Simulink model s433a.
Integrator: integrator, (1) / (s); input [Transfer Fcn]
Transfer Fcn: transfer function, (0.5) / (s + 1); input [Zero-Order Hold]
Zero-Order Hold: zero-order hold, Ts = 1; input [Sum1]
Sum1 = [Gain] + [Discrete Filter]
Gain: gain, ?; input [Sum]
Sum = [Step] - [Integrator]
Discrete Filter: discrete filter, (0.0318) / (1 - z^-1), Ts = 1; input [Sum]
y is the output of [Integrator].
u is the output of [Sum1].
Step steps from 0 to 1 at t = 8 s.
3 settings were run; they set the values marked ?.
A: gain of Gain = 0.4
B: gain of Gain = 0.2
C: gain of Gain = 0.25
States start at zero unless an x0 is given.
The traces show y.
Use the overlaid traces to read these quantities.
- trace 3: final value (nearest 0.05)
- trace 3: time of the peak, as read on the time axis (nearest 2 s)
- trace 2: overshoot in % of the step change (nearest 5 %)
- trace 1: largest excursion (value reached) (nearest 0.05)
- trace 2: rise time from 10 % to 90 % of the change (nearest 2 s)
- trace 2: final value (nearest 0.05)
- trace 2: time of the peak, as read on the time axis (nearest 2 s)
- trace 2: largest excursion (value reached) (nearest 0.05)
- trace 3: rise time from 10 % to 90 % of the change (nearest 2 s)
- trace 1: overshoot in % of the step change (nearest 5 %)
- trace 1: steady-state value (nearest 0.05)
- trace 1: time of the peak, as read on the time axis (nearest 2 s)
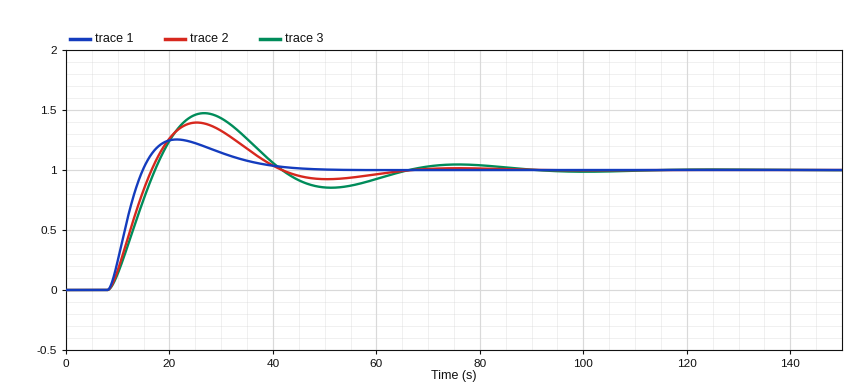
1.00
26 s
40 %
1.25
6 s
1.00
26 s
1.40
6 s
25 %
1.00
22 s
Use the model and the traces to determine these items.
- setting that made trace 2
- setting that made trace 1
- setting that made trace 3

C
A
B
